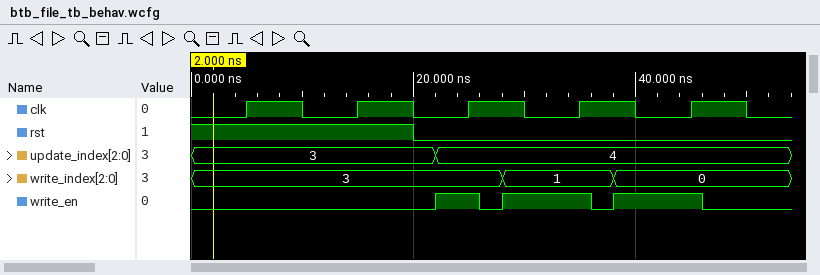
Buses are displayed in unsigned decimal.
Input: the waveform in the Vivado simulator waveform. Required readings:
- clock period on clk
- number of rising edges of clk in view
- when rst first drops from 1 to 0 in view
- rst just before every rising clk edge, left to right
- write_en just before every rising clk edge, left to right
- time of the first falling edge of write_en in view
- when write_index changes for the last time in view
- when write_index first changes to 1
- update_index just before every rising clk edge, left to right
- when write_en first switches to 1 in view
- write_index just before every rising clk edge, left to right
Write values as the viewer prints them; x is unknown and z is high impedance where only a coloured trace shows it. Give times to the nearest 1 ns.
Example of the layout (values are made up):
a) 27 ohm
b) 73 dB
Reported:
a) 10 ns
b) 5
c) 20 ns
d) 1 1 0 0 0
e) 0 0 1 1 1
f) 26 ns
g) 38 ns
h) 28 ns
i) 3, 3, 4, 4, 4
j) 22 ns
k) 3, 3, 3, 1, 0
